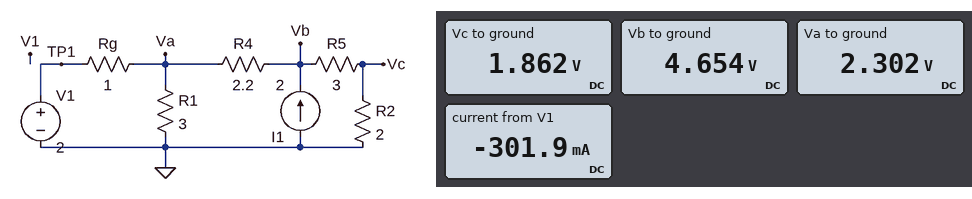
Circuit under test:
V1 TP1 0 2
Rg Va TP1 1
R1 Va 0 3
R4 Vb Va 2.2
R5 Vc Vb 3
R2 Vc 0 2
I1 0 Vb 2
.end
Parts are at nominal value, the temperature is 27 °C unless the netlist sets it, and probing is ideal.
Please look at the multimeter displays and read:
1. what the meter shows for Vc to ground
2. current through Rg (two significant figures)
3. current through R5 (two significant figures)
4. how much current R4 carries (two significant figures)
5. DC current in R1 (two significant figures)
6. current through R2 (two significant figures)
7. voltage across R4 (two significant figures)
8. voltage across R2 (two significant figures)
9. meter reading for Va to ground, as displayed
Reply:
1.862 V
300 mA
930 mA
1.1 A
770 mA
930 mA
2.4 V
1.9 V
2.302 V
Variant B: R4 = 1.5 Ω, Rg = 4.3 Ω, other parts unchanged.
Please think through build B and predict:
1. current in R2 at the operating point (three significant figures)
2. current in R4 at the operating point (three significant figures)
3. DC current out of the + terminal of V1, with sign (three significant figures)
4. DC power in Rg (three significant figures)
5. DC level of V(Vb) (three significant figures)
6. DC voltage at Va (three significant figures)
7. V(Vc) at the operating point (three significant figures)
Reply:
890 mA
1.11 A
-182 mA
143 mW
4.45 V
2.78 V
1.78 V
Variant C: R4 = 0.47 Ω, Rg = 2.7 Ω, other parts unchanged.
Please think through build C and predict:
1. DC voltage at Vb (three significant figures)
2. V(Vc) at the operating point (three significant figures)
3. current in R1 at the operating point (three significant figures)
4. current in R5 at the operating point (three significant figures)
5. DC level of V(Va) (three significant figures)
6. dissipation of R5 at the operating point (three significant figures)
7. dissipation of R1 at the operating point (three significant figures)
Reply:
3.51 V
1.40 V
966 mA
702 mA
2.90 V
1.48 W
2.80 W
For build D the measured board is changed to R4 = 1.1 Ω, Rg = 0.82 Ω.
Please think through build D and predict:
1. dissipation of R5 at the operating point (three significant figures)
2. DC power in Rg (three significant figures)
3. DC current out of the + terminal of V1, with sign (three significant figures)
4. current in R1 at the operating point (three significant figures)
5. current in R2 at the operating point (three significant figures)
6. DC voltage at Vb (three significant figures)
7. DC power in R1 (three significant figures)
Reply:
1.69 W
172 mW
-458 mA
792 mA
750 mA
3.75 V
1.88 W
